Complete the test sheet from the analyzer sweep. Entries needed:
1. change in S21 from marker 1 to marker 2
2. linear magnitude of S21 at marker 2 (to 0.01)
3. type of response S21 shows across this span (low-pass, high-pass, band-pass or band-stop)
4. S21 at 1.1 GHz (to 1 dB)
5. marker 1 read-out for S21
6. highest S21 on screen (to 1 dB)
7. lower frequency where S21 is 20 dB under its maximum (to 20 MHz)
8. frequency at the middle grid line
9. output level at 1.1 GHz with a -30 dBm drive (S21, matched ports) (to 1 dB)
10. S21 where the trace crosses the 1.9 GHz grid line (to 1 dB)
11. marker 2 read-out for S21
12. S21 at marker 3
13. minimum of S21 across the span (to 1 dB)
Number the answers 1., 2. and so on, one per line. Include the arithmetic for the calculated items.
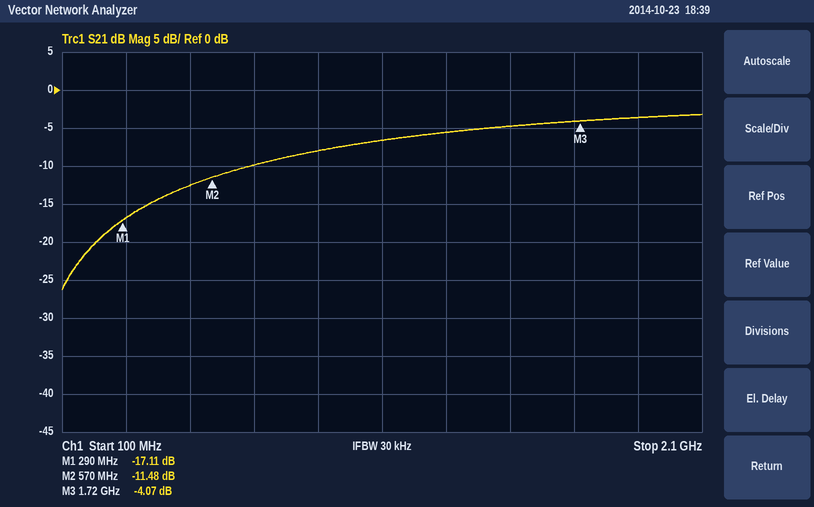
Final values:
1. -11.48 − (-17.11) = 5.63 dB
2. 10^(-11.48/20) ≈ 0.27
3. high-pass
4. -7 dB
5. -17.11 dB
6. -3 dB
7. 140 MHz
8. 1.1 GHz
9. -30 dBm + (-7 dB) = -37 dBm
10. -4 dB
11. -11.48 dB
12. -4.07 dB
13. -26 dB
